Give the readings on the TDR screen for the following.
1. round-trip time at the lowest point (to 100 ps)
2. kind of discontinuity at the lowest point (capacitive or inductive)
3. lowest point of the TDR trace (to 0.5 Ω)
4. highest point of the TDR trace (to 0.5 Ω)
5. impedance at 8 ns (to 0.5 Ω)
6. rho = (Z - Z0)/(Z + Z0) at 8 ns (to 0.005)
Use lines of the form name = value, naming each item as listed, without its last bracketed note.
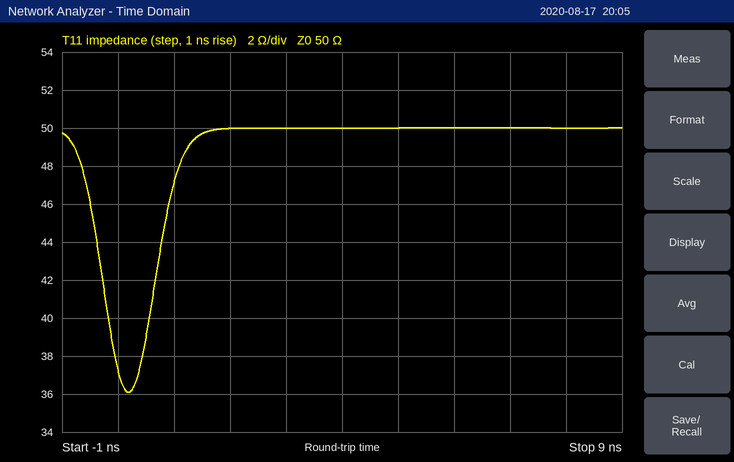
round-trip time at the lowest point = 200 ps
kind of discontinuity at the lowest point = capacitive
lowest point of the TDR trace = 36.0 Ω
highest point of the TDR trace = 50.0 Ω
impedance at 8 ns = 50.0 Ω
rho = (Z - Z0)/(Z + Z0) at 8 ns = 0.000
